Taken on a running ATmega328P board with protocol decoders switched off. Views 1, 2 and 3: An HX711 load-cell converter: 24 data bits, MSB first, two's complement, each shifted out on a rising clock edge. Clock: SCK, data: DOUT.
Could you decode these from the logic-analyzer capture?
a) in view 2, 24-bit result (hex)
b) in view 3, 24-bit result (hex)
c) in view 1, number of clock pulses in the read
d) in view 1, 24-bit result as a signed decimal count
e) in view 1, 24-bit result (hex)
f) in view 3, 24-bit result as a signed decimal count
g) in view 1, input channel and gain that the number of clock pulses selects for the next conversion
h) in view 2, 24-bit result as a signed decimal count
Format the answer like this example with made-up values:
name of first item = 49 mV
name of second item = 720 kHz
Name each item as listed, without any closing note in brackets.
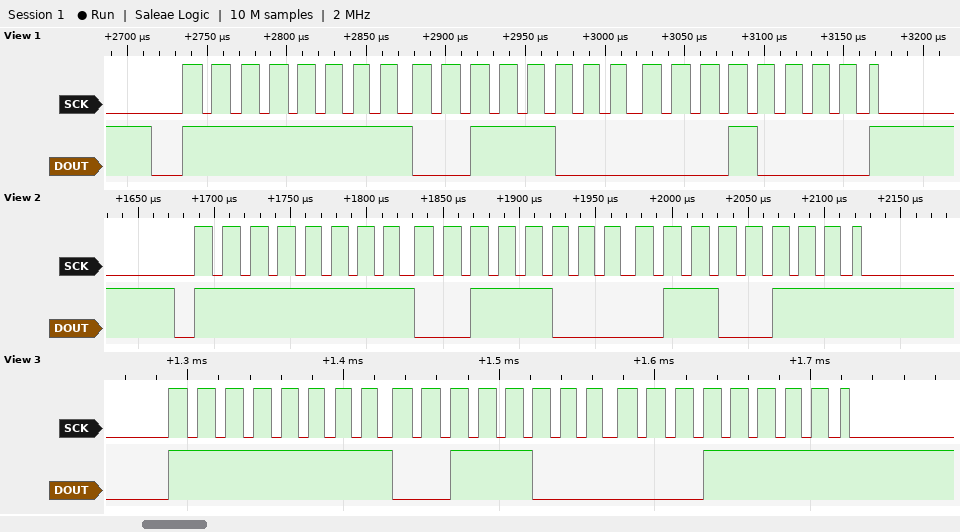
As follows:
in view 2, 24-bit result = 0xFF3867
in view 3, 24-bit result = 0xFF381F
in view 1, number of clock pulses in the read = 25
in view 1, 24-bit result as a signed decimal count = -51184
in view 1, 24-bit result = 0xFF3810
in view 3, 24-bit result as a signed decimal count = -51169
in view 1, input channel and gain that the number of clock pulses selects for the next conversion = channel A, gain 128
in view 2, 24-bit result as a signed decimal count = -51097
